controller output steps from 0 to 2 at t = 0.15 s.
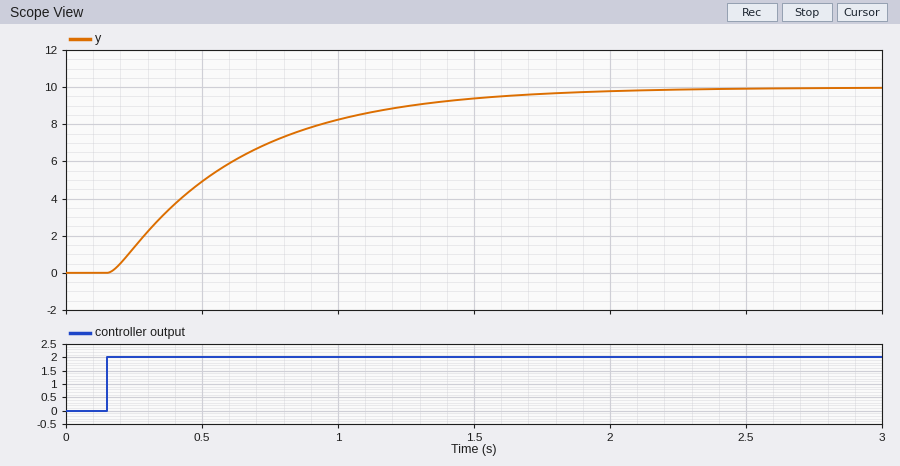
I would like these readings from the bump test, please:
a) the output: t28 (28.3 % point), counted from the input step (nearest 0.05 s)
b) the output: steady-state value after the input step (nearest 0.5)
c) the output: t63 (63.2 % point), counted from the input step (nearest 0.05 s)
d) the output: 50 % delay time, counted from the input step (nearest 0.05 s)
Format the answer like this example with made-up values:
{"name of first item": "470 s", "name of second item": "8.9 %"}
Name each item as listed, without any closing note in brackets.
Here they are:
{"the output: t28 (28.3 % point), counted from the input step": "0.20 s", "the output: steady-state value after the input step": "10.0", "the output: t63 (63.2 % point), counted from the input step": "0.50 s", "the output: 50 % delay time, counted from the input step": "0.35 s"}
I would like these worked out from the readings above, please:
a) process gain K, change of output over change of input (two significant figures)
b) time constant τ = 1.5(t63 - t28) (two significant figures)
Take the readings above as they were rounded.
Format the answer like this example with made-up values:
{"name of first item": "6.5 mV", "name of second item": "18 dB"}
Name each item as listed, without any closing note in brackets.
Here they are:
{"process gain K, change of output over change of input": "5.0", "time constant τ = 1.5(t63 - t28)": "0.45 s"}
